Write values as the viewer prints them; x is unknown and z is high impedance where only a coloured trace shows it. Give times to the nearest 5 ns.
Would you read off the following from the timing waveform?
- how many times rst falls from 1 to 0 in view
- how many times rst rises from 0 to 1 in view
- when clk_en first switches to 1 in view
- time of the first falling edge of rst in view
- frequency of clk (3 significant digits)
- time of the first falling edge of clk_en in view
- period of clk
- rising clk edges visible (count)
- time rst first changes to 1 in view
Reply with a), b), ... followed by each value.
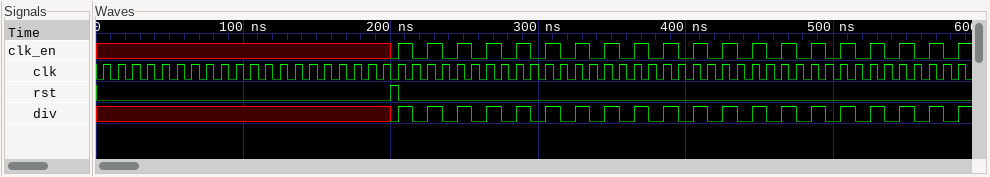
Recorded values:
a) 1
b) 1
c) 205 ns
d) 205 ns
e) 100 MHz
f) 215 ns
g) 10 ns
h) 59
i) 200 ns
